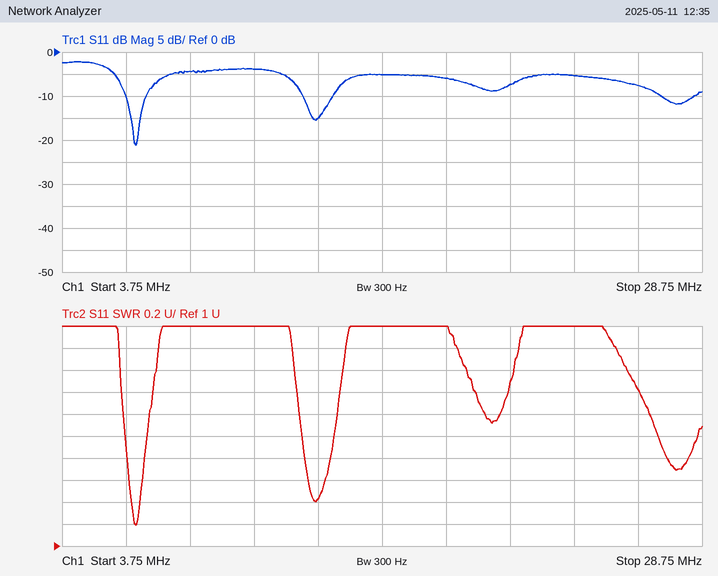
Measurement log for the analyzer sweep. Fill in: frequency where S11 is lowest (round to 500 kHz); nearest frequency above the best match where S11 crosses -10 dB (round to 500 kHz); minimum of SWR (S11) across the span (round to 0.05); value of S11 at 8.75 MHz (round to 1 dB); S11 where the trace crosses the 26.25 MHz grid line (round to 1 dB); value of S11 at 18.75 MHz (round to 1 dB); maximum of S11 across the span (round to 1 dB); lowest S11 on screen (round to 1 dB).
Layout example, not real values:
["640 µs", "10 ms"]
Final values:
["6.5 MHz", "7.0 MHz", "1.20", "-4 dB", "-8 dB", "-6 dB", "-2 dB", "-21 dB"]
